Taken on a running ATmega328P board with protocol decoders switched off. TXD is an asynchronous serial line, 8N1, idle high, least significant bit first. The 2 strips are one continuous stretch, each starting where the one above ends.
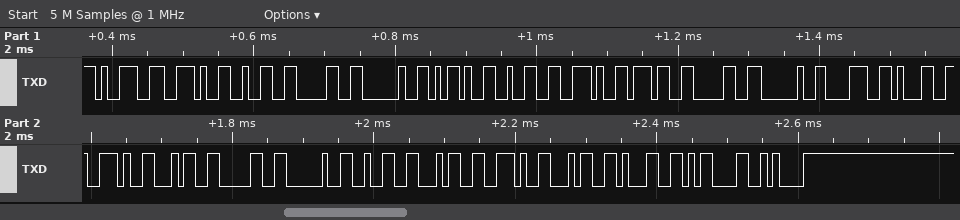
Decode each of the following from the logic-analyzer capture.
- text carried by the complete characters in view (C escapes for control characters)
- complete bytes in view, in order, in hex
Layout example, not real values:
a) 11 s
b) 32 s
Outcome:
a) "9.20 -2.70 81.40 24.41\r\n"
b) 39 2E 32 30 20 2D 32 2E 37 30 20 38 31 2E 34 30 20 32 34 2E 34 31 0D 0A
